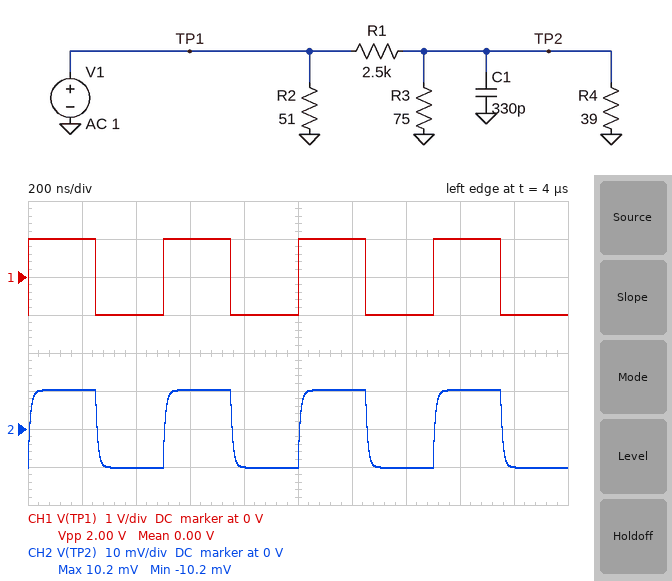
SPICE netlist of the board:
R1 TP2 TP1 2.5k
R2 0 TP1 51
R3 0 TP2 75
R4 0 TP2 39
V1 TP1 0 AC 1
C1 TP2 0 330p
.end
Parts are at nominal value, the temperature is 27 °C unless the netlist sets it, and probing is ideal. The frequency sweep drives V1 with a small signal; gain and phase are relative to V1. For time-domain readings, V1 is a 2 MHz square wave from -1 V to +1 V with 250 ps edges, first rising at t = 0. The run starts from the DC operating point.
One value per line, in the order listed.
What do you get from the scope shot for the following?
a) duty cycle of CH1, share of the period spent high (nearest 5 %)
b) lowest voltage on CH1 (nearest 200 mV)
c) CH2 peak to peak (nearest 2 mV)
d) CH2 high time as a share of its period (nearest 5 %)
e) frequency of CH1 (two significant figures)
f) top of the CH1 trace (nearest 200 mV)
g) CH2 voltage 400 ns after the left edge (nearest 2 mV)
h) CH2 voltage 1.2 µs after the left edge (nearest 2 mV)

50 %
-1.0 V
20 mV
50 %
2.0 MHz
1.0 V
-10 mV
10 mV
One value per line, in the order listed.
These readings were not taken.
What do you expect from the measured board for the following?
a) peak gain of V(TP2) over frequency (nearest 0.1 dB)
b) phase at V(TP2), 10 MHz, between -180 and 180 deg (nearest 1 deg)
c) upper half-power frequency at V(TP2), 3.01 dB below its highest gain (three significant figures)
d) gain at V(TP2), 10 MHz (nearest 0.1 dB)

-39.9 dB
-28 deg
19.0 MHz
-40.9 dB
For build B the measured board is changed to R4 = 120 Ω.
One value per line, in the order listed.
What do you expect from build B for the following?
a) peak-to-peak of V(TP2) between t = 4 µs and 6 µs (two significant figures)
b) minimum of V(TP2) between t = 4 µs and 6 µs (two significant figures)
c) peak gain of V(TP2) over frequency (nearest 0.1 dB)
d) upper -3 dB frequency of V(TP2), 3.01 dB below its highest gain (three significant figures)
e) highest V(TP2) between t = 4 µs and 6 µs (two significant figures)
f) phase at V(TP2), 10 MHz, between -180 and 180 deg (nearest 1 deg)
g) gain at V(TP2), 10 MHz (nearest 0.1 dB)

36 mV
-18 mV
-34.8 dB
10.6 MHz
18 mV
-43 deg
-37.6 dB
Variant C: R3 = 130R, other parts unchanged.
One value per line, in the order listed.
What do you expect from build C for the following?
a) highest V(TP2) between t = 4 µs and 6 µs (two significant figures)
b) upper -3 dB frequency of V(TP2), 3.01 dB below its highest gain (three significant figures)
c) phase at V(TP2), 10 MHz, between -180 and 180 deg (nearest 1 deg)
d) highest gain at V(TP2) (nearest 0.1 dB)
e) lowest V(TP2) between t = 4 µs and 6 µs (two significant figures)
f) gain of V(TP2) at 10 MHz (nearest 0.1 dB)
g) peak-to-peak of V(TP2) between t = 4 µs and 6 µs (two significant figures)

12 mV
16.3 MHz
-32 deg
-38.5 dB
-12 mV
-39.9 dB
24 mV
